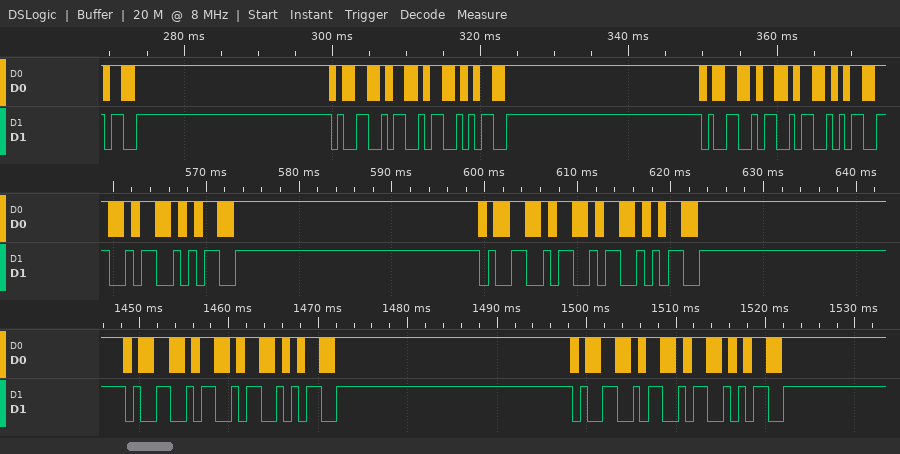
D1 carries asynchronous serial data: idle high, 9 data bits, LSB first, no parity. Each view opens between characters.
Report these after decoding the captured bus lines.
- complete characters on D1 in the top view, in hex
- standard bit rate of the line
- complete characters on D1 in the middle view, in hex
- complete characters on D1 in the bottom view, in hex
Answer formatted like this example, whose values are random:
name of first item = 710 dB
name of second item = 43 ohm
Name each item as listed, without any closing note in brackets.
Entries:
complete characters on D1 in the top view, in hex = 1F3, 99, 9A, 1F3, 99, 9A
standard bit rate of the line = 1200 baud
complete characters on D1 in the middle view, in hex = 9A, 1F3, 99, 9A, 1F3
complete characters on D1 in the bottom view, in hex = 99, 9A, 1F3, 99, 9A, 1F3
